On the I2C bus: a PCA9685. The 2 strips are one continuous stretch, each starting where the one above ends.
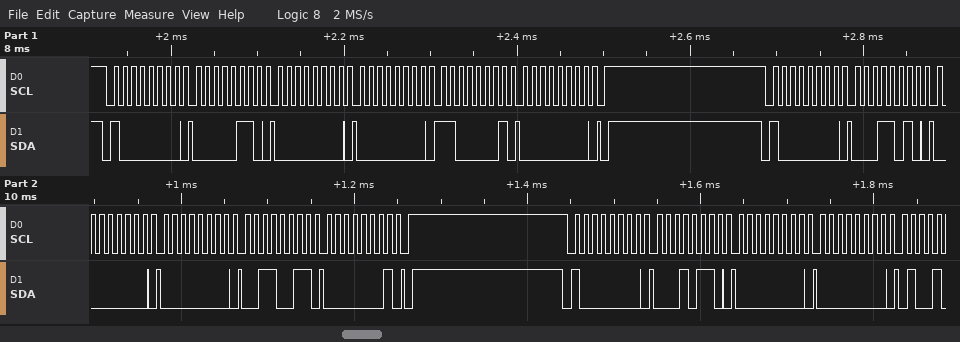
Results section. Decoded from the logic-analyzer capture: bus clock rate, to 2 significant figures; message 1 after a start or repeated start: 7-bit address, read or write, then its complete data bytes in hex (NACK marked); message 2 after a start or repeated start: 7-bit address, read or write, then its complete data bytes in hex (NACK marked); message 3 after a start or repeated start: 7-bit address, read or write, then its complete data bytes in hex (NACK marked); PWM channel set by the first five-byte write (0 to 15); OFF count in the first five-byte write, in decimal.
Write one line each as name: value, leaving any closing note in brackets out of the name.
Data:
bus clock rate, to 2 significant figures: 100 kHz
message 1 after a start or repeated start: 7-bit address, read or write, then its complete data bytes in hex: 0x40 write: 06 00 00 C1 00
message 2 after a start or repeated start: 7-bit address, read or write, then its complete data bytes in hex: 0x40 write: 1A 00 00 33 01
message 3 after a start or repeated start: 7-bit address, read or write, then its complete data bytes in hex: 0x40 write: 16 00 00
PWM channel set by the first five-byte write: 0
OFF count in the first five-byte write, in decimal: 193
